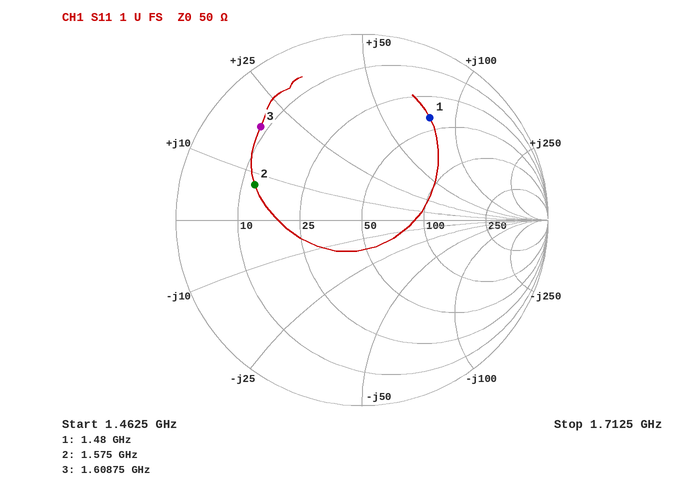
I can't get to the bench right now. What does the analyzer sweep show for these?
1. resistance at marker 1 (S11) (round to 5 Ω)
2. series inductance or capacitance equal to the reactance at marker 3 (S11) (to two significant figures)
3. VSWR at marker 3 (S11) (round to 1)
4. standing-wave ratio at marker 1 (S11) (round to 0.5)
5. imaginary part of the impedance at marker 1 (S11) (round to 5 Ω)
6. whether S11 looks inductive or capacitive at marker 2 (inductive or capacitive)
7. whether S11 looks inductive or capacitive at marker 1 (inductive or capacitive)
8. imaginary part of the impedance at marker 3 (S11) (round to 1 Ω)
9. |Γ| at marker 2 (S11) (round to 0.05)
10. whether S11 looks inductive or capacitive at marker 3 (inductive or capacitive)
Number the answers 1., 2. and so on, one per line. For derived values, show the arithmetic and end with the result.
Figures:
1. 40 Ω
2. L = 19 Ω/(2π × 1.60875 GHz) ≈ 1.9 nH
3. 7
4. 5.0
5. +80 Ω
6. inductive
7. inductive
8. +19 Ω
9. 0.60
10. inductive
